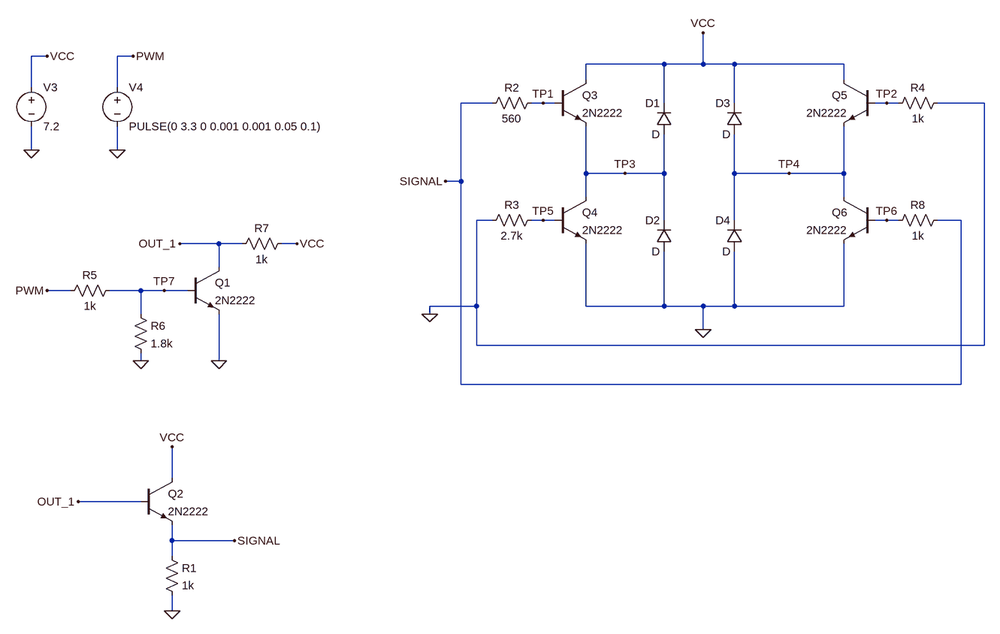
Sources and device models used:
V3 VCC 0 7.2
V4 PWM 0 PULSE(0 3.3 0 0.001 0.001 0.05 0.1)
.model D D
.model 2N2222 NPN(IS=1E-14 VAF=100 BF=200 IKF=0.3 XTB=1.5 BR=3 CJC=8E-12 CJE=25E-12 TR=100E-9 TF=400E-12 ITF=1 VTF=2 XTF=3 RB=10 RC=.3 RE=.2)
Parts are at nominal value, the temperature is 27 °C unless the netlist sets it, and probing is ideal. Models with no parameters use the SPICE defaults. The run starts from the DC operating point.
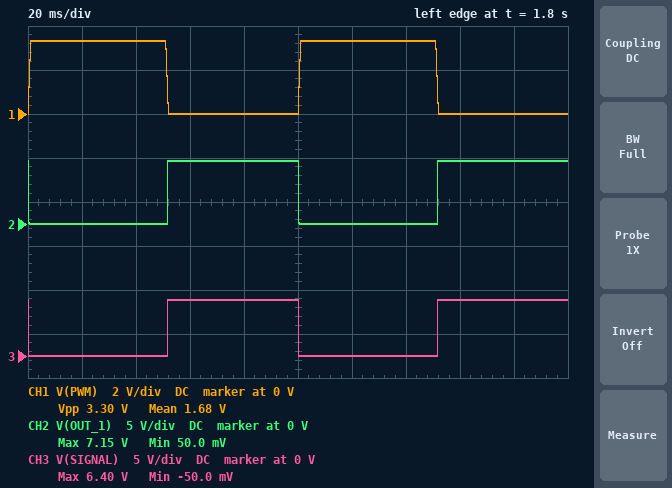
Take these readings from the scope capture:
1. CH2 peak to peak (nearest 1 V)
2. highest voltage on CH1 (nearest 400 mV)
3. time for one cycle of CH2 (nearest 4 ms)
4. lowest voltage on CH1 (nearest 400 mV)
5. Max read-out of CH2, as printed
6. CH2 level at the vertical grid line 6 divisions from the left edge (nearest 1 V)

7 V
3.2 V
100 ms
0 V
7.15 V
0 V
